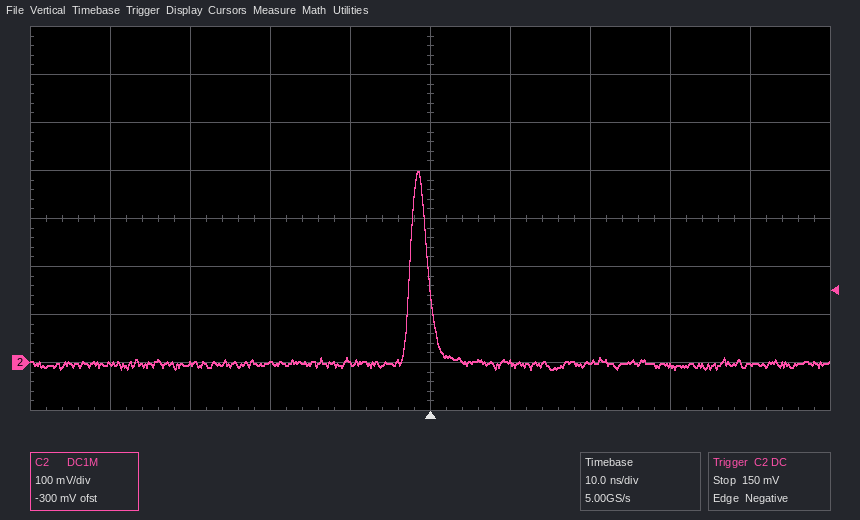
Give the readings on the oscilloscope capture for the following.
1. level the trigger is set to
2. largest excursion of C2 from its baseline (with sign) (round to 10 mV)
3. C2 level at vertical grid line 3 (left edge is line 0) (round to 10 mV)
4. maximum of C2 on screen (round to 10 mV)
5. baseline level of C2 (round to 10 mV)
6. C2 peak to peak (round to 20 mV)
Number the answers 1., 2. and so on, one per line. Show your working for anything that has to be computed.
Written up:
1. 150 mV
2. 400 mV − (0 mV) = +400 mV
3. 0 mV
4. 400 mV
5. 0 mV
6. 420 mV
